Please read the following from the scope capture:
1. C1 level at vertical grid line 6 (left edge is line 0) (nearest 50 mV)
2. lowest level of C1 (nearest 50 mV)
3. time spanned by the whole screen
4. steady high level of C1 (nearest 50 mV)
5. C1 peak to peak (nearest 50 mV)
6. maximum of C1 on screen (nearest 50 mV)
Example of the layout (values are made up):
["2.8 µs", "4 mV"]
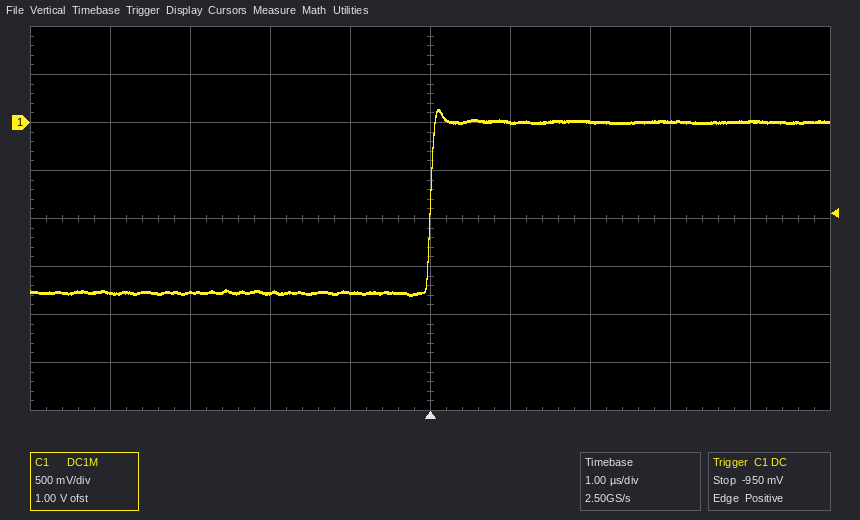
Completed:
["0 mV", "-1.80 V", "10 µs", "0 mV", "1.95 V", "150 mV"]
